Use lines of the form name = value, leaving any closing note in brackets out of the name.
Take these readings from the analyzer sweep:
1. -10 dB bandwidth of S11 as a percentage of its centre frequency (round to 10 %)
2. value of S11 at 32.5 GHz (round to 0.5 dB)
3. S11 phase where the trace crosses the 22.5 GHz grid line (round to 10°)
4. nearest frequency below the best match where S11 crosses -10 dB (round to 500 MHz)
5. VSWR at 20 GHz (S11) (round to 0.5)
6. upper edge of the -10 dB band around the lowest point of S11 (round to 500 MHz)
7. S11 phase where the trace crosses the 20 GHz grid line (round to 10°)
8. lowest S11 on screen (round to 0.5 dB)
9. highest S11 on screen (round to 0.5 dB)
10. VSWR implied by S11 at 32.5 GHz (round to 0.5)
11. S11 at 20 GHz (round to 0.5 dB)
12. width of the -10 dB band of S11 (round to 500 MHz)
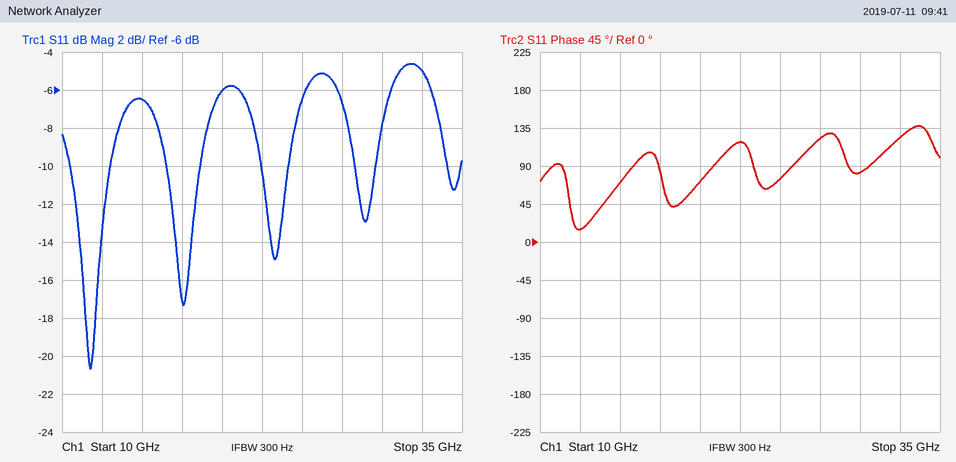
-10 dB bandwidth of S11 as a percentage of its centre frequency = 20 %
value of S11 at 32.5 GHz = -5.0 dB
S11 phase where the trace crosses the 22.5 GHz grid line = 120°
nearest frequency below the best match where S11 crosses -10 dB = 10.5 GHz
VSWR at 20 GHz (S11) = 3.0
upper edge of the -10 dB band around the lowest point of S11 = 13.0 GHz
S11 phase where the trace crosses the 20 GHz grid line = 70°
lowest S11 on screen = -20.5 dB
highest S11 on screen = -4.5 dB
VSWR implied by S11 at 32.5 GHz = 3.5
S11 at 20 GHz = -6.0 dB
width of the -10 dB band of S11 = 2.5 GHz
